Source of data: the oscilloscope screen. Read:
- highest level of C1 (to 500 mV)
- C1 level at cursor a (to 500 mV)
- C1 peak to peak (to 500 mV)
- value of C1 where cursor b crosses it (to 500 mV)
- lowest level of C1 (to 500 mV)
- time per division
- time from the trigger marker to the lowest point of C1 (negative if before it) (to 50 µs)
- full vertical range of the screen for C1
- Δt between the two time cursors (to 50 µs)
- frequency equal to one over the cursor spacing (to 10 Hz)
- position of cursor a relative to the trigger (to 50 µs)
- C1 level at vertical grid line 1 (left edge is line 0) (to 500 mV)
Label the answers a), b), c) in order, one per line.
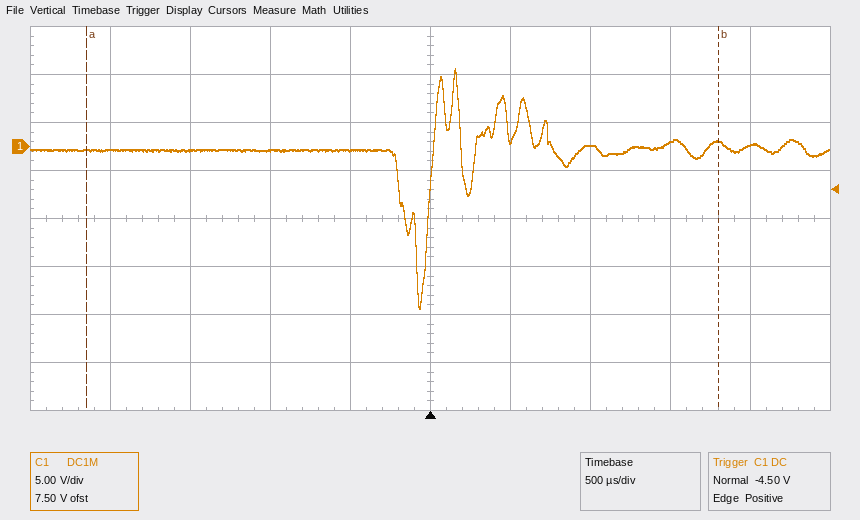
a) 8.0 V
b) -500 mV
c) 25.0 V
d) 500 mV
e) -17.0 V
f) 500 µs
g) -50 µs
h) 40 V
i) 3.95 ms
j) 250 Hz
k) -2.15 ms
l) -500 mV
